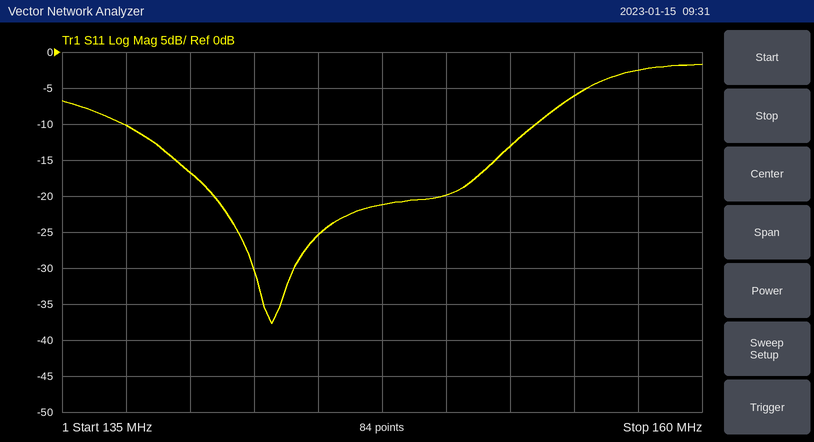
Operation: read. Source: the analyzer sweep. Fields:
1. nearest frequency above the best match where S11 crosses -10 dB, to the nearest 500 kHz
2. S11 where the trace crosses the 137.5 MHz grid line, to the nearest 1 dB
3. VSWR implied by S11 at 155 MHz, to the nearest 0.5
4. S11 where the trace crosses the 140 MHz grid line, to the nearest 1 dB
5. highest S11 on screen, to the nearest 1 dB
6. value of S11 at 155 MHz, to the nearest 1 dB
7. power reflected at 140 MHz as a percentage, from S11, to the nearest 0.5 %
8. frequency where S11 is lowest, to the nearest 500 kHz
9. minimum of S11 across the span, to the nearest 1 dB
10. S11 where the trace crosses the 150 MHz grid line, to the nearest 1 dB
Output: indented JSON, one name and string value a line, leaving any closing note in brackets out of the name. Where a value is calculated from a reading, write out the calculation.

{
  "nearest frequency above the best match where S11 crosses -10 dB, to the nearest 500 kHz": "153.5 MHz",
  "S11 where the trace crosses the 137.5 MHz grid line, to the nearest 1 dB": "-10 dB",
  "VSWR implied by S11 at 155 MHz, to the nearest 0.5": "|Γ| = 10^(-6/20) = 0.5012; VSWR = (1 + 0.5012)/(1 − 0.5012) ≈ 3.0",
  "S11 where the trace crosses the 140 MHz grid line, to the nearest 1 dB": "-17 dB",
  "highest S11 on screen, to the nearest 1 dB": "-2 dB",
  "value of S11 at 155 MHz, to the nearest 1 dB": "-6 dB",
  "power reflected at 140 MHz as a percentage, from S11, to the nearest 0.5 %": "10^(-17/10) ≈ 2.0 %",
  "frequency where S11 is lowest, to the nearest 500 kHz": "143.0 MHz",
  "minimum of S11 across the span, to the nearest 1 dB": "-38 dB",
  "S11 where the trace crosses the 150 MHz grid line, to the nearest 1 dB": "-20 dB"
}
